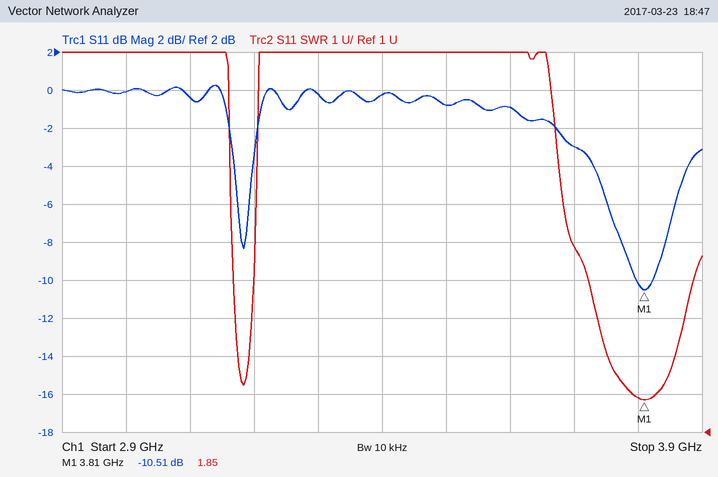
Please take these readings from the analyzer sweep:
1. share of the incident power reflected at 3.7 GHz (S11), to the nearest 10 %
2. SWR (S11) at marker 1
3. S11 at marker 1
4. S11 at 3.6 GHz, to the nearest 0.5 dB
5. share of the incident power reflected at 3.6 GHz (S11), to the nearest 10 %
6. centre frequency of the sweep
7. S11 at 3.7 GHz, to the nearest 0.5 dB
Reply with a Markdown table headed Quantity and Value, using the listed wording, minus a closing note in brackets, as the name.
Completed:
| Quantity | Value |
|---|---|
| share of the incident power reflected at 3.7 GHz (S11), to the nearest 10 % | 50 % |
| SWR (S11) at marker 1 | 1.85 |
| S11 at marker 1 | -10.51 dB |
| S11 at 3.6 GHz, to the nearest 0.5 dB | -1.0 dB |
| share of the incident power reflected at 3.6 GHz (S11), to the nearest 10 % | 80 % |
| centre frequency of the sweep | 3.4 GHz |
| S11 at 3.7 GHz, to the nearest 0.5 dB | -3.0 dB |
